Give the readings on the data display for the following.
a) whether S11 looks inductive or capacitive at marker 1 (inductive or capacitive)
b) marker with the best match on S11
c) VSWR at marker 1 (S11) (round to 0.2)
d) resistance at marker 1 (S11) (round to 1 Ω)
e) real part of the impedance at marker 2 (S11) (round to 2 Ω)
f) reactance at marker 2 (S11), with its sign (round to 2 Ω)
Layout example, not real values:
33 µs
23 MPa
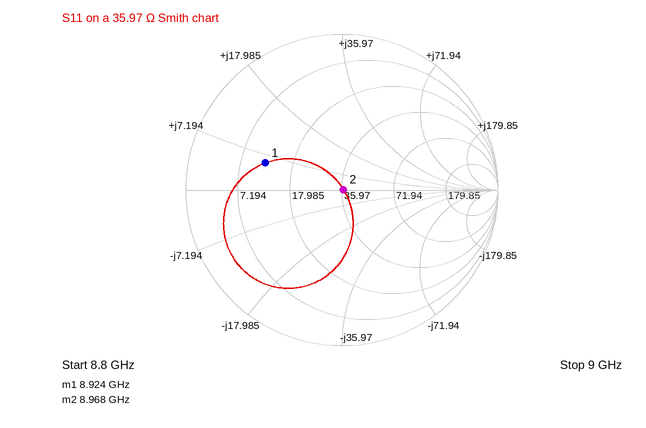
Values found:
inductive
marker 2
3.2
12 Ω
36 Ω
0 Ω
